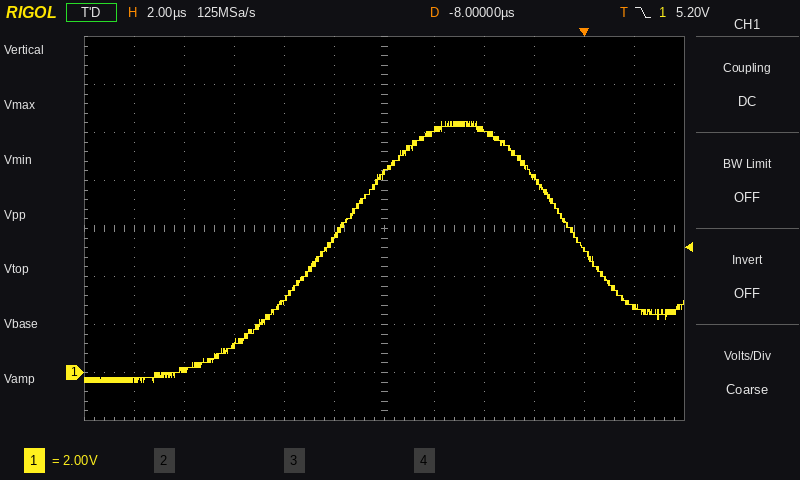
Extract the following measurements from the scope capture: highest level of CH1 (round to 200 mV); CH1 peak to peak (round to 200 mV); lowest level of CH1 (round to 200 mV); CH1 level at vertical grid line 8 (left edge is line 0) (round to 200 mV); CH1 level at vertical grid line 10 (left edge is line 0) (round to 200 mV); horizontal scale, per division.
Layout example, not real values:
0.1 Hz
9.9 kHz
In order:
10.4 V
10.8 V
-400 mV
10.2 V
5.2 V
2 µs
